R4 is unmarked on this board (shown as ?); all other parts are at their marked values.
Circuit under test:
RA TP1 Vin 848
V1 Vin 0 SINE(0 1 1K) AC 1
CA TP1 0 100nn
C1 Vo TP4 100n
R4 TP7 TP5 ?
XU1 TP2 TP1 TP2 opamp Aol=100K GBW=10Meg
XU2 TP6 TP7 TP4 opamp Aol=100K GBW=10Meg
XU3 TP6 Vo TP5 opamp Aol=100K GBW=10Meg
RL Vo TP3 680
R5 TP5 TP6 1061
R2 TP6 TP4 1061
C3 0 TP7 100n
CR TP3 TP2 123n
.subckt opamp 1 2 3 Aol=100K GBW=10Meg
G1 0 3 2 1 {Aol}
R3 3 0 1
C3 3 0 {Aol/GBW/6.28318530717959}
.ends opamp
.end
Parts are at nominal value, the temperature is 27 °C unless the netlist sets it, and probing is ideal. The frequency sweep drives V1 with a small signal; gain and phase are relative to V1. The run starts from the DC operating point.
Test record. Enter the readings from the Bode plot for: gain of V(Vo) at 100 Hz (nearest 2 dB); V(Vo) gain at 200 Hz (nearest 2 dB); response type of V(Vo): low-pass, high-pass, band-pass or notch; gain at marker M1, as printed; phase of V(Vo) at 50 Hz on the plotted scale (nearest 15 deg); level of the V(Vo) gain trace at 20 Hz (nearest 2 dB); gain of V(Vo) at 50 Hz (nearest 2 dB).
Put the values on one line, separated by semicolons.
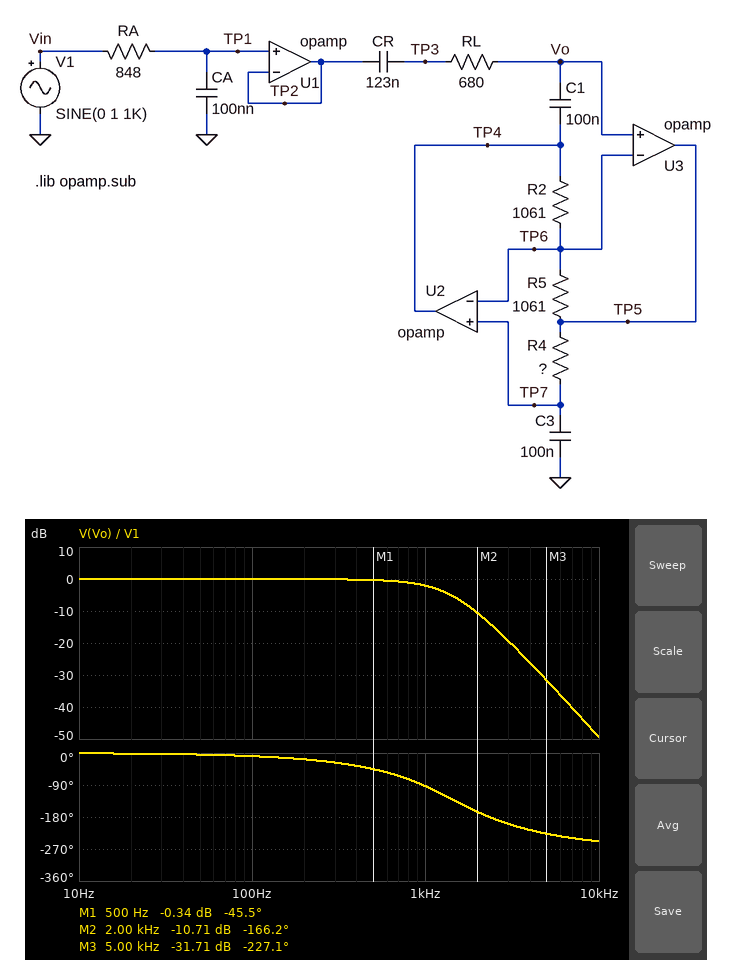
0 dB; 0 dB; low-pass; -0.34 dB; 0 deg; 0 dB; 0 dB
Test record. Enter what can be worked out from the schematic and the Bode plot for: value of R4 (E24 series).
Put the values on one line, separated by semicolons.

2 kΩ
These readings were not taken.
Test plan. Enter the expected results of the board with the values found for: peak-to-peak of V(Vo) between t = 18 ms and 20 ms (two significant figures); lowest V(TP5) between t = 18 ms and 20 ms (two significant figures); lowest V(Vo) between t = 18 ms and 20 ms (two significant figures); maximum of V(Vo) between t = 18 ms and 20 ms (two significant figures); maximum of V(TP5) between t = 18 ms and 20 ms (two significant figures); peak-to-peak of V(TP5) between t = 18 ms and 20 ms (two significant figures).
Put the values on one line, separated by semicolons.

1.6 V; -1.3 V; -790 mV; 790 mV; 1.3 V; 2.5 V
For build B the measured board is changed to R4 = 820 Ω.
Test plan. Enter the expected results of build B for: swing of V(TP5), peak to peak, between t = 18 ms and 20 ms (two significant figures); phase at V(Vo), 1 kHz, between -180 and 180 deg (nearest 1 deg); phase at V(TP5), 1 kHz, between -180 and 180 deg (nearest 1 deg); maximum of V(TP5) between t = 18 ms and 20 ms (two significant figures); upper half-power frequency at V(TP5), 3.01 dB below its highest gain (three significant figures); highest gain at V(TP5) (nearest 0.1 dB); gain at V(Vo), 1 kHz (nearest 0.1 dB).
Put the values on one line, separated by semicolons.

2.2 V; -56 deg; -29 deg; 1.1 V; 2.51 kHz; 1.8 dB; 0 dB
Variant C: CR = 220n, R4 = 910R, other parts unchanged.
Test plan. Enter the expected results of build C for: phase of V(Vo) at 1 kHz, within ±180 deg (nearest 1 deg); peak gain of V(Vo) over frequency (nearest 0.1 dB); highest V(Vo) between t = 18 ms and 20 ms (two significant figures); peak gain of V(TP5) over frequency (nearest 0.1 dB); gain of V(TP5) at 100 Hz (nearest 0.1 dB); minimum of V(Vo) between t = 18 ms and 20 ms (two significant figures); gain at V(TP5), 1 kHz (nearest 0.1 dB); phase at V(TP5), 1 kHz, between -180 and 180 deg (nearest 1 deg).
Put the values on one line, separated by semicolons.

-47 deg; 3.0 dB; 1.1 V; 6.2 dB; 0 dB; -1.1 V; 2.1 dB; -17 deg
